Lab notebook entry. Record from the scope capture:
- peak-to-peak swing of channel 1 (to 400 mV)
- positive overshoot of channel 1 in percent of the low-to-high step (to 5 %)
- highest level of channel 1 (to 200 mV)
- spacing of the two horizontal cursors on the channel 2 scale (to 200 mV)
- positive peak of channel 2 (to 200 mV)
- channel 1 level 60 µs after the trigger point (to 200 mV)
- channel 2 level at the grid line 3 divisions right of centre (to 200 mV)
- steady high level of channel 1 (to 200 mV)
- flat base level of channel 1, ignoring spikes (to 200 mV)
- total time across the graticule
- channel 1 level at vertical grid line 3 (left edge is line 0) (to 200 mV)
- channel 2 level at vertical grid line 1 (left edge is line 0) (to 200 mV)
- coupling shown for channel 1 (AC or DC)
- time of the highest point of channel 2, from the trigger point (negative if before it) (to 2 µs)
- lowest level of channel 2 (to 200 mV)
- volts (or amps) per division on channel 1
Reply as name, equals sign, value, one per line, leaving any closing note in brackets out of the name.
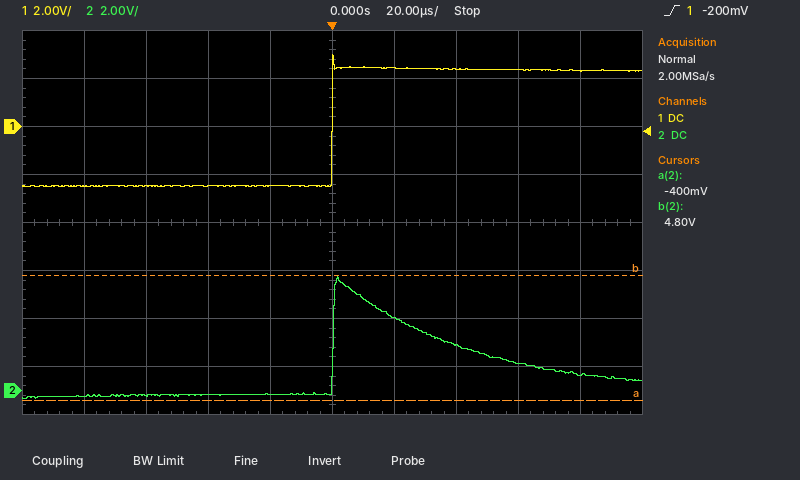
peak-to-peak swing of channel 1 = 5.6 V
positive overshoot of channel 1 in percent of the low-to-high step = 15 %
highest level of channel 1 = 3.0 V
spacing of the two horizontal cursors on the channel 2 scale = 5.2 V
positive peak of channel 2 = 4.8 V
channel 1 level 60 µs after the trigger point = 2.4 V
channel 2 level at the grid line 3 divisions right of centre = 1.2 V
steady high level of channel 1 = 2.4 V
flat base level of channel 1, ignoring spikes = -2.4 V
total time across the graticule = 200 µs
channel 1 level at vertical grid line 3 (left edge is line 0) = -2.4 V
channel 2 level at vertical grid line 1 (left edge is line 0) = -200 mV
coupling shown for channel 1 = DC
time of the highest point of channel 2, from the trigger point (negative if before it) = +2 µs
lowest level of channel 2 = -400 mV
volts (or amps) per division on channel 1 = 2 V
